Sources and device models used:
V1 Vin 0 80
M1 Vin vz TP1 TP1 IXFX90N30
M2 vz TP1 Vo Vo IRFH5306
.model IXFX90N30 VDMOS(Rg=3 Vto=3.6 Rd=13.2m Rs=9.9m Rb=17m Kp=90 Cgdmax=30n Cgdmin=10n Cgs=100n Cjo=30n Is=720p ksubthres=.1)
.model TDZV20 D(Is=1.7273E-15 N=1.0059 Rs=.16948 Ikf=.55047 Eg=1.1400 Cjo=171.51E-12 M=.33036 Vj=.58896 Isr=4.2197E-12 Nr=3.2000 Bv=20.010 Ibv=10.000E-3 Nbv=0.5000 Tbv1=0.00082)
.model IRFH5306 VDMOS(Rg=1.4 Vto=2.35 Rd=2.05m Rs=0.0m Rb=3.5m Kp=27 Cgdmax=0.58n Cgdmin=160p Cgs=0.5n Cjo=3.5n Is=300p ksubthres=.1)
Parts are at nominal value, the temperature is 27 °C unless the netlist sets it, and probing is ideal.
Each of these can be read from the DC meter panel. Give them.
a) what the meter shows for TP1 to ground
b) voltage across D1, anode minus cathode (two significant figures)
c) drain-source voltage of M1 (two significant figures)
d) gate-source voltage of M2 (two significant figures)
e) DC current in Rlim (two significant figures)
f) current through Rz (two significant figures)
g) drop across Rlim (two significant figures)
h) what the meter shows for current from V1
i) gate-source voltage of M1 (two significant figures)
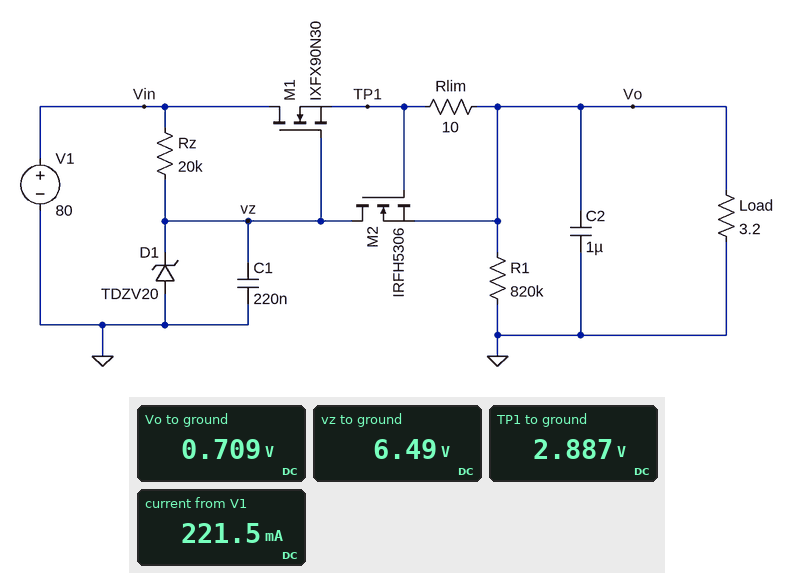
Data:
2.887 V
-6.5 V
77 V
2.2 V
220 mA
3.7 mA
2.2 V
221.5 mA
3.6 V
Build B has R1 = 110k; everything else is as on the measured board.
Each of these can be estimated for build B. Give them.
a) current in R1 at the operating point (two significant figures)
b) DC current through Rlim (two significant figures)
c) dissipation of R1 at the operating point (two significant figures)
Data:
6.4 µA
220 mA
4.6 µW
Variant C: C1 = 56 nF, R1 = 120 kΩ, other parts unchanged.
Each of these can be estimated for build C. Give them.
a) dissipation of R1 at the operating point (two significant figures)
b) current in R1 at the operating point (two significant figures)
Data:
4.2 µW
5.9 µA
